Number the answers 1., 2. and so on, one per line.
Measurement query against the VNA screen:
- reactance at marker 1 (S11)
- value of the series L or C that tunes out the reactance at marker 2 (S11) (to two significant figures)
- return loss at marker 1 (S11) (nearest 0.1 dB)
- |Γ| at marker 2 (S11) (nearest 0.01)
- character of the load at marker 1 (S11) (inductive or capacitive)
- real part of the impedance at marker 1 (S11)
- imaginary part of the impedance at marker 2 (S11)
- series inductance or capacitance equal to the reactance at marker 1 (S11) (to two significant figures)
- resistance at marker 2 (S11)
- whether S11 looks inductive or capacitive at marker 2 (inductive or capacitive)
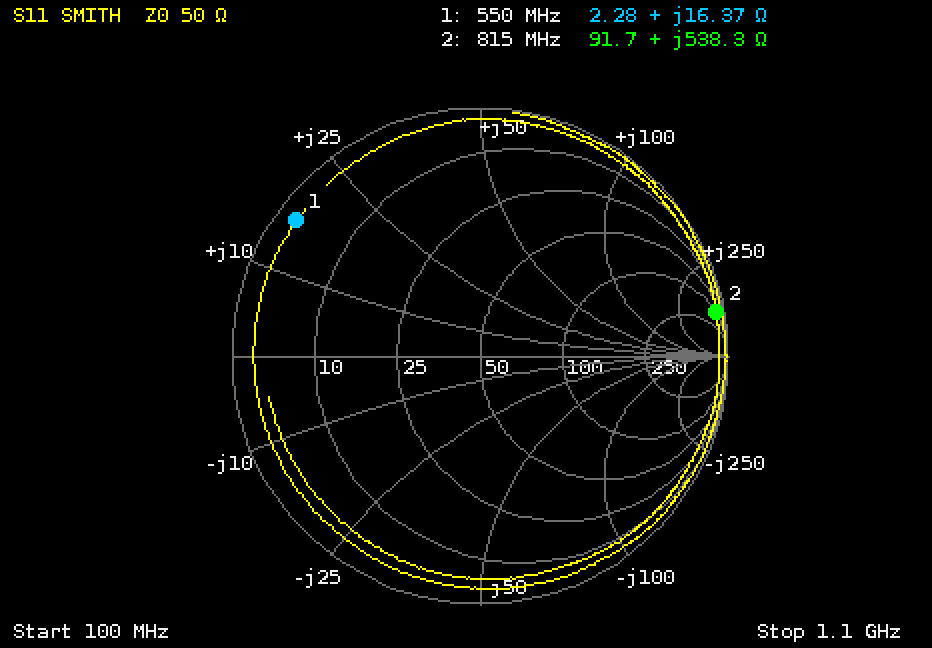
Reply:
1. +16.37 Ω
2. 360 fF
3. 0.7 dB
4. 0.97
5. inductive
6. 2.28 Ω
7. +538.3 Ω
8. 4.7 nH
9. 91.7 Ω
10. inductive
